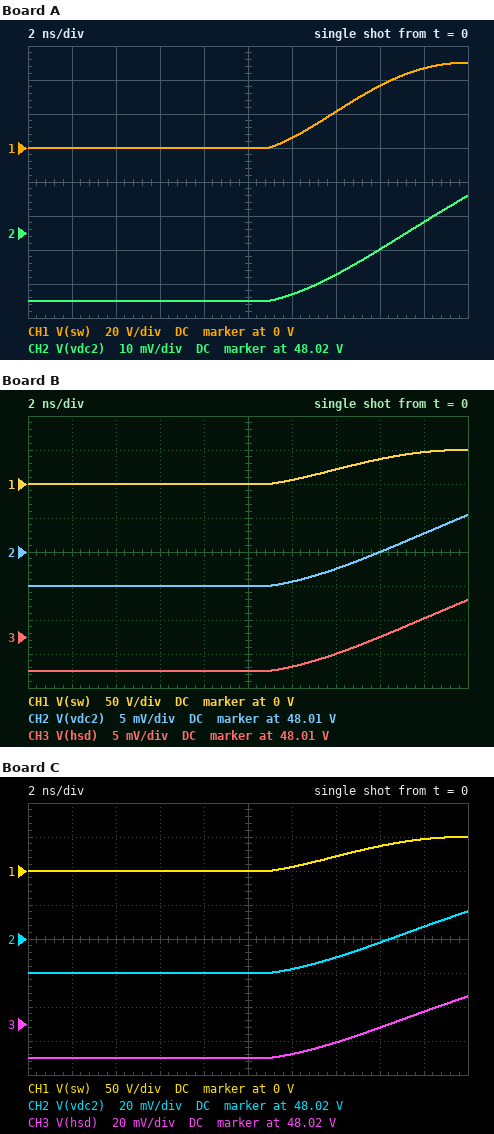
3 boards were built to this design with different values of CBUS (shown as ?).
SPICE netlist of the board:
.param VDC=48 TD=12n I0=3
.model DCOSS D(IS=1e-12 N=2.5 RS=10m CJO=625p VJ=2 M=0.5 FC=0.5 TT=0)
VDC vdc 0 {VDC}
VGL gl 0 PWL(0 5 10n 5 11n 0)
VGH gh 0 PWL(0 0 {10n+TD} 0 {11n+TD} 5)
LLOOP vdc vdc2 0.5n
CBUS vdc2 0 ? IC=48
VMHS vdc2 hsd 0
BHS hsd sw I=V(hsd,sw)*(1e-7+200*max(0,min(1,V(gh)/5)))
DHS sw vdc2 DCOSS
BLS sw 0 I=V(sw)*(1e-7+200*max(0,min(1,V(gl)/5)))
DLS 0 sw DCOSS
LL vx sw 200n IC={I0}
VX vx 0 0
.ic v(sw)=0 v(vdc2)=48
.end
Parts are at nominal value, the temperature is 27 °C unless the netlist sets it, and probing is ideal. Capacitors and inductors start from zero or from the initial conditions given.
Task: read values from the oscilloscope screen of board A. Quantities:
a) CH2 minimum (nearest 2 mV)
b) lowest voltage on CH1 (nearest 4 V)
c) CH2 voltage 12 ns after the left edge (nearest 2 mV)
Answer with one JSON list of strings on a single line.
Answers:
["48.000 V", "0 V", "48.002 V"]
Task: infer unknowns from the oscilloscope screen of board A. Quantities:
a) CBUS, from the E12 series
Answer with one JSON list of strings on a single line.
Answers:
["390 nF"]
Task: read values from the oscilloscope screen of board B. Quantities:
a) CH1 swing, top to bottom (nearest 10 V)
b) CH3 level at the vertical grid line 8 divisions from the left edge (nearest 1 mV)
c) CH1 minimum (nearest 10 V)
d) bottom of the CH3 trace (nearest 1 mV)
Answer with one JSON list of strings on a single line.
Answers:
["50 V", "48.005 V", "0 V", "48.000 V"]
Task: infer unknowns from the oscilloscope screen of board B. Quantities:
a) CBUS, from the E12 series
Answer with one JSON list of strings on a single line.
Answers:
["1.2 µF"]
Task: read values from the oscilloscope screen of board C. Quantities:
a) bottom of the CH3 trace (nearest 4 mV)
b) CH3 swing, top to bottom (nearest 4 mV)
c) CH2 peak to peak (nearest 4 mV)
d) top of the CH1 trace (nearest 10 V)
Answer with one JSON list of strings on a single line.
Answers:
["48.000 V", "36 mV", "36 mV", "50 V"]
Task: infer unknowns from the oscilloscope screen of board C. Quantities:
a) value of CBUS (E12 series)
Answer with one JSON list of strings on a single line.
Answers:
["330 nF"]
